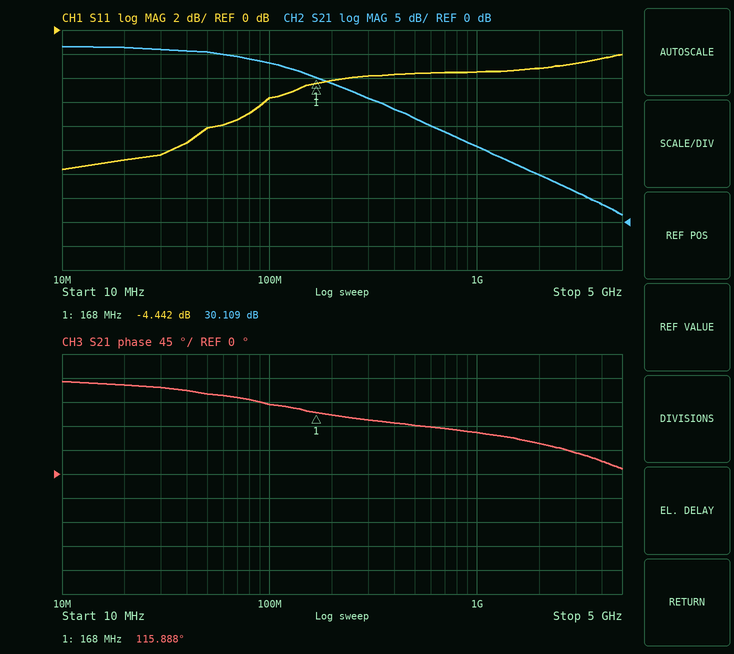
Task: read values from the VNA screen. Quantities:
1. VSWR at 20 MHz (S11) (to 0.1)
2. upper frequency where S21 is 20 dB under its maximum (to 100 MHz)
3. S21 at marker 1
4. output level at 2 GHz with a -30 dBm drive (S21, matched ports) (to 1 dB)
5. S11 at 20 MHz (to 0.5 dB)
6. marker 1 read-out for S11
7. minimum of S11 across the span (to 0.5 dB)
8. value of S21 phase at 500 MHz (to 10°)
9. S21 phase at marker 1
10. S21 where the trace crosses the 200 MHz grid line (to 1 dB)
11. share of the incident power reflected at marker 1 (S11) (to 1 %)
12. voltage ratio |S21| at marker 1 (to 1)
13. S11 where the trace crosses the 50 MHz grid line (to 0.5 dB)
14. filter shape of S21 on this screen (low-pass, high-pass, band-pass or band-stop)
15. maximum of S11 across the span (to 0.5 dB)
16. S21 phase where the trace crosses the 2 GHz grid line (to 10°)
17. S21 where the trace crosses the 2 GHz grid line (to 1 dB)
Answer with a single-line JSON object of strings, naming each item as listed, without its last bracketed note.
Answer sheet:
{"VSWR at 20 MHz (S11)": "1.8", "upper frequency where S21 is 20 dB under its maximum": "900 MHz", "S21 at marker 1": "30.109 dB", "output level at 2 GHz with a -30 dBm drive (S21, matched ports)": "-20 dBm", "S11 at 20 MHz": "-11.0 dB", "marker 1 read-out for S11": "-4.442 dB", "minimum of S11 across the span": "-11.5 dB", "value of S21 phase at 500 MHz": "90°", "S21 phase at marker 1": "115.888°", "S21 where the trace crosses the 200 MHz grid line": "29 dB", "share of the incident power reflected at marker 1 (S11)": "36 %", "voltage ratio |S21| at marker 1": "32", "S11 where the trace crosses the 50 MHz grid line": "-8.0 dB", "filter shape of S21 on this screen": "low-pass", "maximum of S11 across the span": "-2.0 dB", "S21 phase where the trace crosses the 2 GHz grid line": "60°", "S21 where the trace crosses the 2 GHz grid line": "10 dB"}
